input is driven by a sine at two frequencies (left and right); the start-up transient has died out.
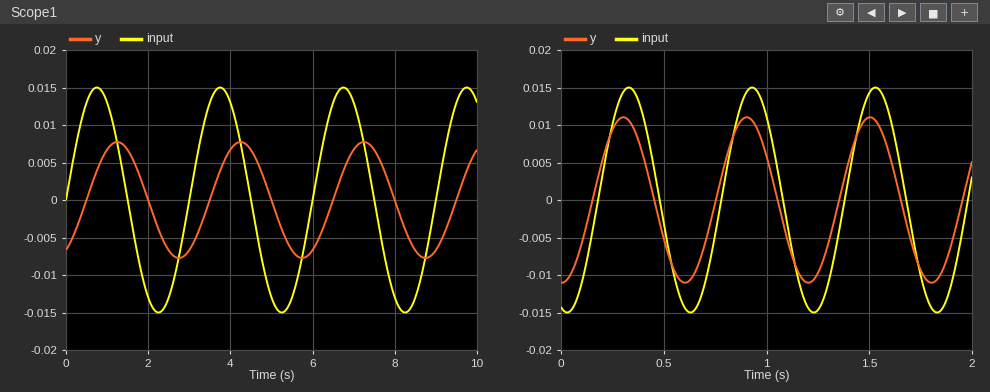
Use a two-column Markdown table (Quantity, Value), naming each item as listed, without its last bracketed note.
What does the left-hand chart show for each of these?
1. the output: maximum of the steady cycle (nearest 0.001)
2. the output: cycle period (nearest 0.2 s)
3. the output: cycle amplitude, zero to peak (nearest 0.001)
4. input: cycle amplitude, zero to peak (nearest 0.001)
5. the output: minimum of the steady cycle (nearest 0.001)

| Quantity | Value |
|---|---|
| the output: maximum of the steady cycle | 0.008 |
| the output: cycle period | 3.0 s |
| the output: cycle amplitude, zero to peak | 0.008 |
| input: cycle amplitude, zero to peak | 0.015 |
| the output: minimum of the steady cycle | -0.008 |
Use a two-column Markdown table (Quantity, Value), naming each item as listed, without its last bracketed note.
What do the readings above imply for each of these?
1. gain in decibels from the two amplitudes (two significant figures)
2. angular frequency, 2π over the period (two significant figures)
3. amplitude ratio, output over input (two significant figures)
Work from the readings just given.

| Quantity | Value |
|---|---|
| gain in decibels from the two amplitudes | -5.5 dB |
| angular frequency, 2π over the period | 2.1 rad/s |
| amplitude ratio, output over input | 0.53 |
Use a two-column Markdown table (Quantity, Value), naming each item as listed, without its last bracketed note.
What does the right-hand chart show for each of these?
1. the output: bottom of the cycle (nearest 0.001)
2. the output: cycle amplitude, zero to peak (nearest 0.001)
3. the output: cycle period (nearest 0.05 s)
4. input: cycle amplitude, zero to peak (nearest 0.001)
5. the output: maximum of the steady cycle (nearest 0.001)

| Quantity | Value |
|---|---|
| the output: bottom of the cycle | -0.011 |
| the output: cycle amplitude, zero to peak | 0.011 |
| the output: cycle period | 0.60 s |
| input: cycle amplitude, zero to peak | 0.015 |
| the output: maximum of the steady cycle | 0.011 |
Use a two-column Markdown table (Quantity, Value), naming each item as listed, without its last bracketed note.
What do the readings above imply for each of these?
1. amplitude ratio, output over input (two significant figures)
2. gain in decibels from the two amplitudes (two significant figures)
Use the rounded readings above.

| Quantity | Value |
|---|---|
| amplitude ratio, output over input | 0.73 |
| gain in decibels from the two amplitudes | -2.7 dB |
